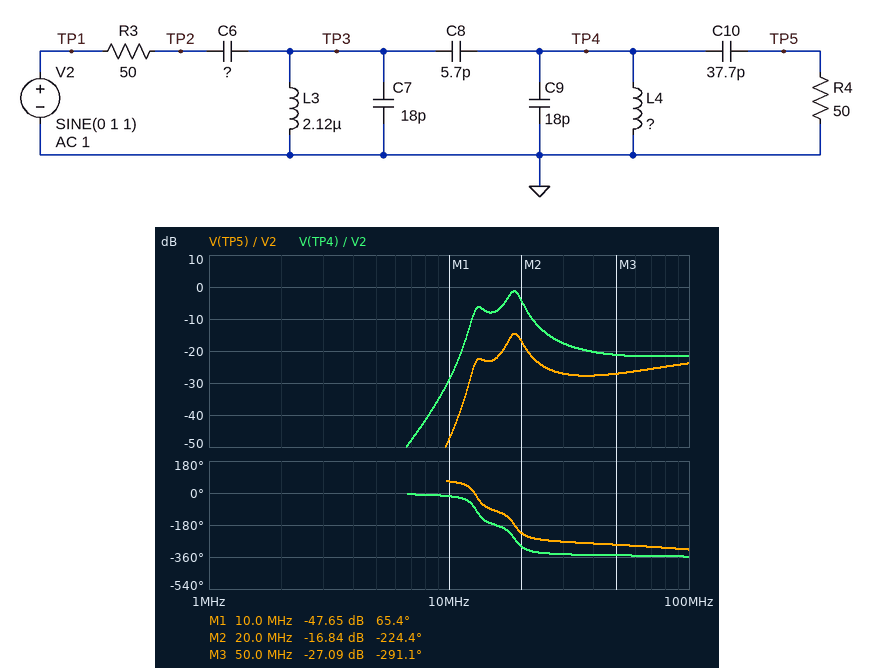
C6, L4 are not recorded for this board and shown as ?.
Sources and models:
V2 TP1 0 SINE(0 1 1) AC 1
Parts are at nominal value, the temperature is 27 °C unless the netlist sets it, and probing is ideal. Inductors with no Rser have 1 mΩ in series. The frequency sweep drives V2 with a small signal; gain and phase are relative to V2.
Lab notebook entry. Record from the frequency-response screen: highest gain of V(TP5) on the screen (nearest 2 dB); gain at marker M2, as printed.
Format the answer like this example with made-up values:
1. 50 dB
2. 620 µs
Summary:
1. -14 dB
2. -16.84 dB
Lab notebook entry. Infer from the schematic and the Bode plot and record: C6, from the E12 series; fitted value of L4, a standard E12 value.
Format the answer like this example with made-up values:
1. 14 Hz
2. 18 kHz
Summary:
1. 47 pF
2. 1.2 µH
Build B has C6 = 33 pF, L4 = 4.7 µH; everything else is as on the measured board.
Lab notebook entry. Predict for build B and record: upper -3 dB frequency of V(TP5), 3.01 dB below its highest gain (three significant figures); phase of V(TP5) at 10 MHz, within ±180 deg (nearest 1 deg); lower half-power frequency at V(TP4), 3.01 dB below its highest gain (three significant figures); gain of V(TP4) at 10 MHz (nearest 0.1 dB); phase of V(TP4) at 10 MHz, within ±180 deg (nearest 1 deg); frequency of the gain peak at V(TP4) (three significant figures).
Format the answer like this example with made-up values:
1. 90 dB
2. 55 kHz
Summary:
1. 15.4 MHz
2. -75 deg
3. 14.0 MHz
4. -9.4 dB
5. -158 deg
6. 14.7 MHz
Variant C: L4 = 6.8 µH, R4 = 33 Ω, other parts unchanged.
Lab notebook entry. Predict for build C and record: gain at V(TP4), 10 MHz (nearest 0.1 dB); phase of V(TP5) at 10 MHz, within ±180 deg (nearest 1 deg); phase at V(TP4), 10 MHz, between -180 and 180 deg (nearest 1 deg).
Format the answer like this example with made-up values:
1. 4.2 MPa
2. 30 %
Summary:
1. -13.4 dB
2. -104 deg
3. 171 deg
